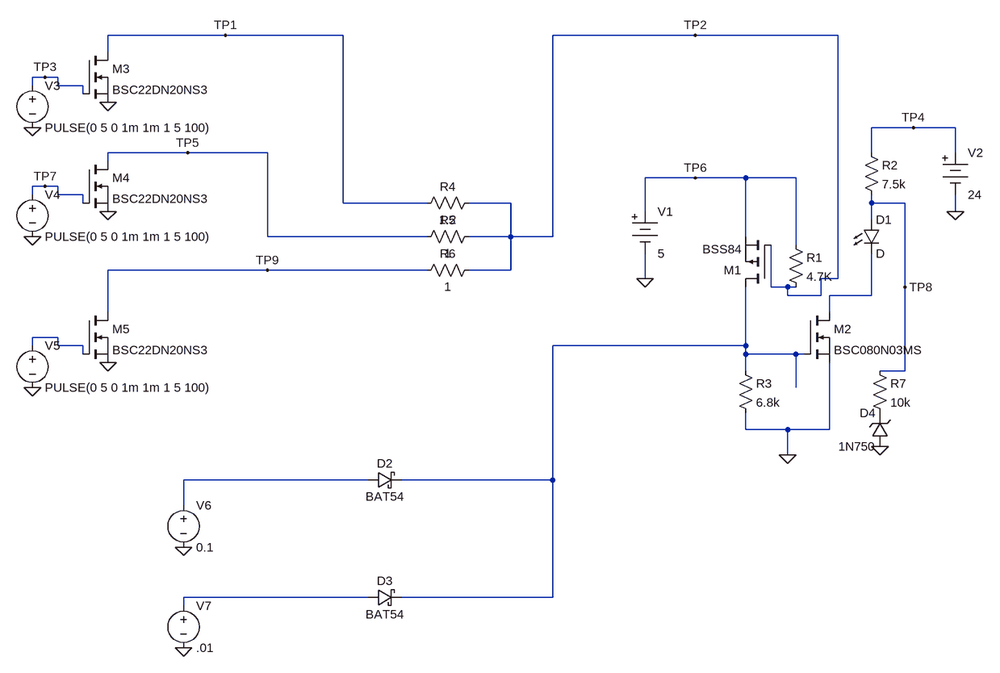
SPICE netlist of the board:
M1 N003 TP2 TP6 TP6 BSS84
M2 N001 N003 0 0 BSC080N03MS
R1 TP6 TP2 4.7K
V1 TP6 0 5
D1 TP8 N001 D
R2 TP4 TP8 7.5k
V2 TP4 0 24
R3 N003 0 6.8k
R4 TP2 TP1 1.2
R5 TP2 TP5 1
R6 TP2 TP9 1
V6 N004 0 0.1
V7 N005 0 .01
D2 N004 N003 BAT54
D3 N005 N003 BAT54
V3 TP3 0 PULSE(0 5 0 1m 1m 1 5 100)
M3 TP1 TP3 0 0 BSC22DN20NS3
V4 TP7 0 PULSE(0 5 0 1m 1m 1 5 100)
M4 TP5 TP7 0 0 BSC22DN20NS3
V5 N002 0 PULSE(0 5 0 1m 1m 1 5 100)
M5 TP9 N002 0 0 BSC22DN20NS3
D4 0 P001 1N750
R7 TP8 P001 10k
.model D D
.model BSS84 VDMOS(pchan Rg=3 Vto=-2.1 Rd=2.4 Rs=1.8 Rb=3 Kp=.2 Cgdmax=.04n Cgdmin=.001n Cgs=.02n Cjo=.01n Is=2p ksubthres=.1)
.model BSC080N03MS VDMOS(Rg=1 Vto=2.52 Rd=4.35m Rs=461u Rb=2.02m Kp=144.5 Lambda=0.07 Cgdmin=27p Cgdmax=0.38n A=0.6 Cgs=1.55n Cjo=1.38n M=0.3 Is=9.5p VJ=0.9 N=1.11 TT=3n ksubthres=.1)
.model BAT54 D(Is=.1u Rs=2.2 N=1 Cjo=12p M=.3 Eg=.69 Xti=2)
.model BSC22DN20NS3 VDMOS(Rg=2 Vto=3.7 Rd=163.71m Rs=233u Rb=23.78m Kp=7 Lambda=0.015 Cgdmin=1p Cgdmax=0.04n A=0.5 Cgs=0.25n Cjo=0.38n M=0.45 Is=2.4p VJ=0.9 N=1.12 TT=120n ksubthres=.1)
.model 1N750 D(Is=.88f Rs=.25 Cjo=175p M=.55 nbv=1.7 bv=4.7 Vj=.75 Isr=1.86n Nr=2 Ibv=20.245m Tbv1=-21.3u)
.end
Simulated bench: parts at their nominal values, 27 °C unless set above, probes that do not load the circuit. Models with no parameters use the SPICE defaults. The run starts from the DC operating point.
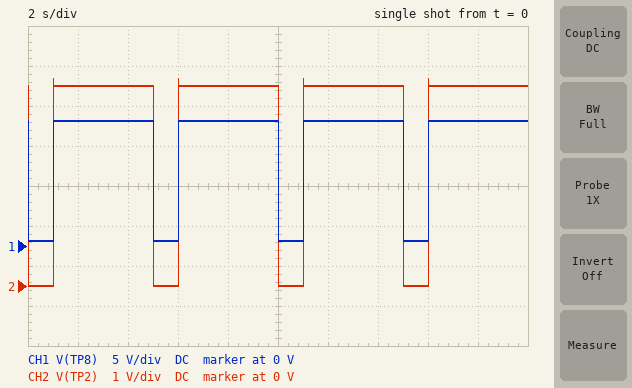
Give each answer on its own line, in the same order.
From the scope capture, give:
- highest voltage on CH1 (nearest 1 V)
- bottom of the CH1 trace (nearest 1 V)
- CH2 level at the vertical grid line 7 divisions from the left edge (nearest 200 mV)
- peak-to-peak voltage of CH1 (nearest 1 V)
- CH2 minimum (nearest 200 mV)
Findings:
16 V
1 V
5.0 V
15 V
0 V
